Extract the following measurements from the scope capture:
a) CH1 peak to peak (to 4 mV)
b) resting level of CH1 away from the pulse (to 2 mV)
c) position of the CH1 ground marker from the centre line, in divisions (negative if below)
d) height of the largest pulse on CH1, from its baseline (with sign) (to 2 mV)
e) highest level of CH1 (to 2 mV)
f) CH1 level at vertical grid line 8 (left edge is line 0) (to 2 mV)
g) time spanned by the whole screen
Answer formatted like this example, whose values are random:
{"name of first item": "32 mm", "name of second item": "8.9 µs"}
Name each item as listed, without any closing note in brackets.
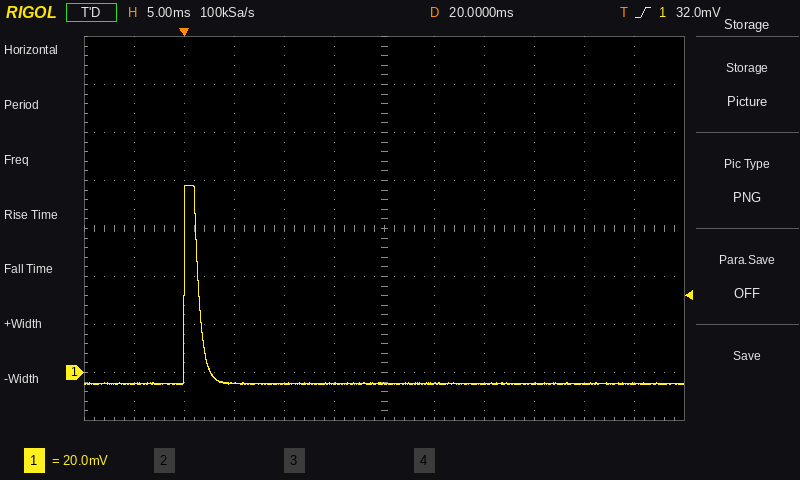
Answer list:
{"CH1 peak to peak": "84 mV", "resting level of CH1 away from the pulse": "-4 mV", "position of the CH1 ground marker from the centre line, in divisions": "-3.0 div", "height of the largest pulse on CH1, from its baseline (with sign)": "+82 mV", "highest level of CH1": "78 mV", "CH1 level at vertical grid line 8 (left edge is line 0)": "-4 mV", "time spanned by the whole screen": "60 ms"}
